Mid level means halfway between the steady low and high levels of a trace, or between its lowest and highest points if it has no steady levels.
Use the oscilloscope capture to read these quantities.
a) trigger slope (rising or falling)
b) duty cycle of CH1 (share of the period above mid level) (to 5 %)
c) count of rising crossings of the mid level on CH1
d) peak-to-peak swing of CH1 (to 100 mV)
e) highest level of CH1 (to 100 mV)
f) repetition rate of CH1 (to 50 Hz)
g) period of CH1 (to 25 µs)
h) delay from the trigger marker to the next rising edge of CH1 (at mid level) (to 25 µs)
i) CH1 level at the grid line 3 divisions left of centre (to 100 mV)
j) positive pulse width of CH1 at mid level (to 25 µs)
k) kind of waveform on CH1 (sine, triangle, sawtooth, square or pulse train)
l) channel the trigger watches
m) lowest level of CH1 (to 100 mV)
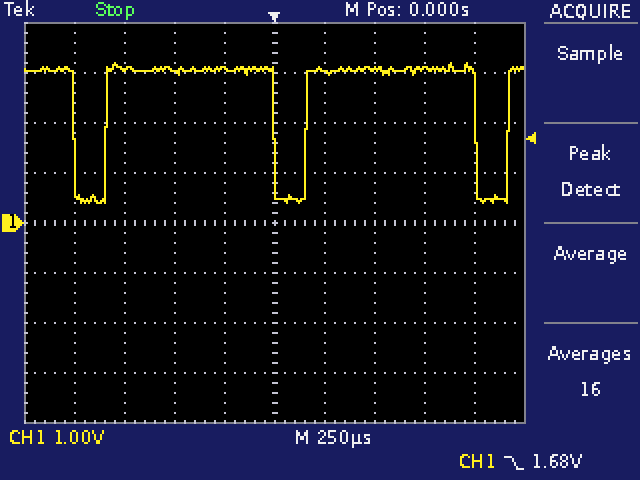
falling
85 %
3
2.8 V
3.2 V
1.00 kHz
1.000 ms
150 µs
3.1 V
850 µs
pulse train
CH1
400 mV
